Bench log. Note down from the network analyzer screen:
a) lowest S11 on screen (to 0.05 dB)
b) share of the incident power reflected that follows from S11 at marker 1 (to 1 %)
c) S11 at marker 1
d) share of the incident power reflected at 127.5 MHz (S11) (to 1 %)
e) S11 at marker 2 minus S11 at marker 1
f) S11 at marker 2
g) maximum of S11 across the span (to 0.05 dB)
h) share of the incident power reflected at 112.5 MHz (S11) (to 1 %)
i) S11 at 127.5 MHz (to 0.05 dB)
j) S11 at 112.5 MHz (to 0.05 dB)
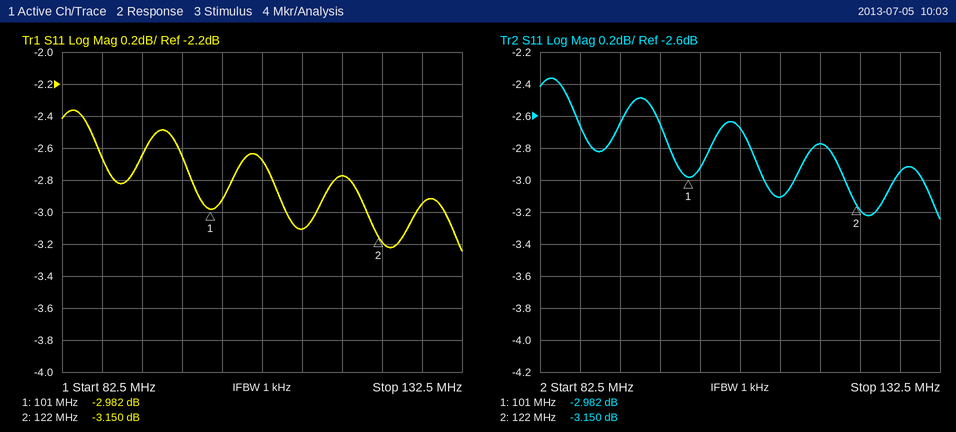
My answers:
-3.25 dB
50 %
-2.982 dB
51 %
-0.168 dB
-3.150 dB
-2.35 dB
49 %
-2.95 dB
-3.10 dB
